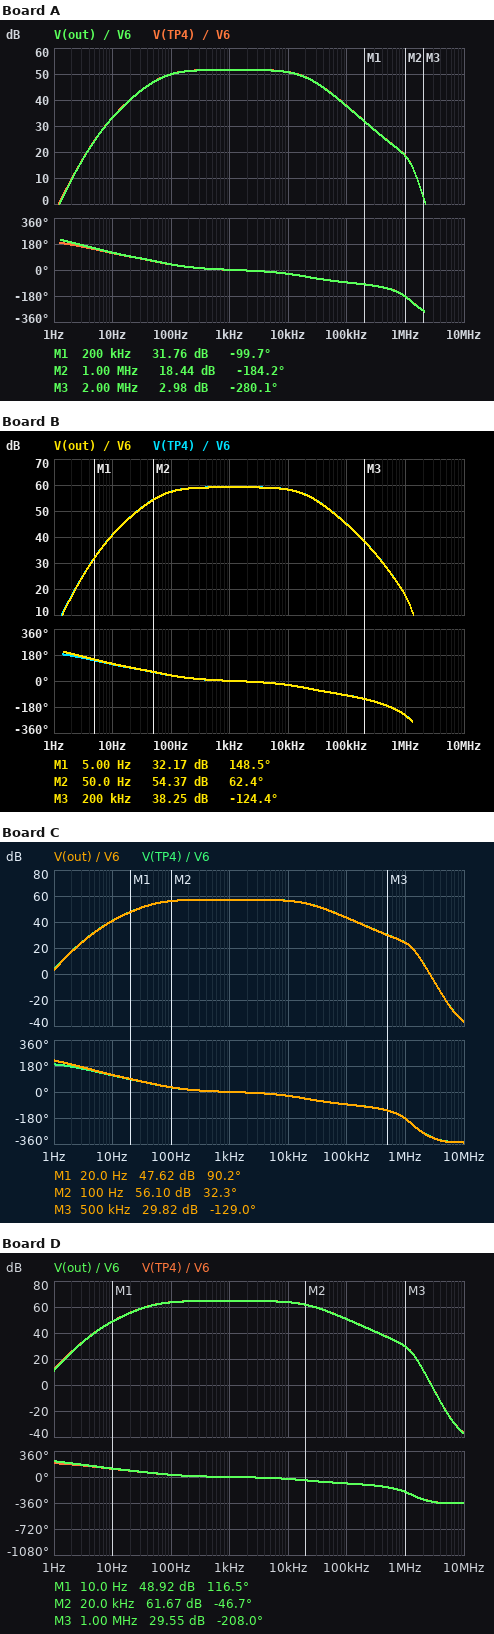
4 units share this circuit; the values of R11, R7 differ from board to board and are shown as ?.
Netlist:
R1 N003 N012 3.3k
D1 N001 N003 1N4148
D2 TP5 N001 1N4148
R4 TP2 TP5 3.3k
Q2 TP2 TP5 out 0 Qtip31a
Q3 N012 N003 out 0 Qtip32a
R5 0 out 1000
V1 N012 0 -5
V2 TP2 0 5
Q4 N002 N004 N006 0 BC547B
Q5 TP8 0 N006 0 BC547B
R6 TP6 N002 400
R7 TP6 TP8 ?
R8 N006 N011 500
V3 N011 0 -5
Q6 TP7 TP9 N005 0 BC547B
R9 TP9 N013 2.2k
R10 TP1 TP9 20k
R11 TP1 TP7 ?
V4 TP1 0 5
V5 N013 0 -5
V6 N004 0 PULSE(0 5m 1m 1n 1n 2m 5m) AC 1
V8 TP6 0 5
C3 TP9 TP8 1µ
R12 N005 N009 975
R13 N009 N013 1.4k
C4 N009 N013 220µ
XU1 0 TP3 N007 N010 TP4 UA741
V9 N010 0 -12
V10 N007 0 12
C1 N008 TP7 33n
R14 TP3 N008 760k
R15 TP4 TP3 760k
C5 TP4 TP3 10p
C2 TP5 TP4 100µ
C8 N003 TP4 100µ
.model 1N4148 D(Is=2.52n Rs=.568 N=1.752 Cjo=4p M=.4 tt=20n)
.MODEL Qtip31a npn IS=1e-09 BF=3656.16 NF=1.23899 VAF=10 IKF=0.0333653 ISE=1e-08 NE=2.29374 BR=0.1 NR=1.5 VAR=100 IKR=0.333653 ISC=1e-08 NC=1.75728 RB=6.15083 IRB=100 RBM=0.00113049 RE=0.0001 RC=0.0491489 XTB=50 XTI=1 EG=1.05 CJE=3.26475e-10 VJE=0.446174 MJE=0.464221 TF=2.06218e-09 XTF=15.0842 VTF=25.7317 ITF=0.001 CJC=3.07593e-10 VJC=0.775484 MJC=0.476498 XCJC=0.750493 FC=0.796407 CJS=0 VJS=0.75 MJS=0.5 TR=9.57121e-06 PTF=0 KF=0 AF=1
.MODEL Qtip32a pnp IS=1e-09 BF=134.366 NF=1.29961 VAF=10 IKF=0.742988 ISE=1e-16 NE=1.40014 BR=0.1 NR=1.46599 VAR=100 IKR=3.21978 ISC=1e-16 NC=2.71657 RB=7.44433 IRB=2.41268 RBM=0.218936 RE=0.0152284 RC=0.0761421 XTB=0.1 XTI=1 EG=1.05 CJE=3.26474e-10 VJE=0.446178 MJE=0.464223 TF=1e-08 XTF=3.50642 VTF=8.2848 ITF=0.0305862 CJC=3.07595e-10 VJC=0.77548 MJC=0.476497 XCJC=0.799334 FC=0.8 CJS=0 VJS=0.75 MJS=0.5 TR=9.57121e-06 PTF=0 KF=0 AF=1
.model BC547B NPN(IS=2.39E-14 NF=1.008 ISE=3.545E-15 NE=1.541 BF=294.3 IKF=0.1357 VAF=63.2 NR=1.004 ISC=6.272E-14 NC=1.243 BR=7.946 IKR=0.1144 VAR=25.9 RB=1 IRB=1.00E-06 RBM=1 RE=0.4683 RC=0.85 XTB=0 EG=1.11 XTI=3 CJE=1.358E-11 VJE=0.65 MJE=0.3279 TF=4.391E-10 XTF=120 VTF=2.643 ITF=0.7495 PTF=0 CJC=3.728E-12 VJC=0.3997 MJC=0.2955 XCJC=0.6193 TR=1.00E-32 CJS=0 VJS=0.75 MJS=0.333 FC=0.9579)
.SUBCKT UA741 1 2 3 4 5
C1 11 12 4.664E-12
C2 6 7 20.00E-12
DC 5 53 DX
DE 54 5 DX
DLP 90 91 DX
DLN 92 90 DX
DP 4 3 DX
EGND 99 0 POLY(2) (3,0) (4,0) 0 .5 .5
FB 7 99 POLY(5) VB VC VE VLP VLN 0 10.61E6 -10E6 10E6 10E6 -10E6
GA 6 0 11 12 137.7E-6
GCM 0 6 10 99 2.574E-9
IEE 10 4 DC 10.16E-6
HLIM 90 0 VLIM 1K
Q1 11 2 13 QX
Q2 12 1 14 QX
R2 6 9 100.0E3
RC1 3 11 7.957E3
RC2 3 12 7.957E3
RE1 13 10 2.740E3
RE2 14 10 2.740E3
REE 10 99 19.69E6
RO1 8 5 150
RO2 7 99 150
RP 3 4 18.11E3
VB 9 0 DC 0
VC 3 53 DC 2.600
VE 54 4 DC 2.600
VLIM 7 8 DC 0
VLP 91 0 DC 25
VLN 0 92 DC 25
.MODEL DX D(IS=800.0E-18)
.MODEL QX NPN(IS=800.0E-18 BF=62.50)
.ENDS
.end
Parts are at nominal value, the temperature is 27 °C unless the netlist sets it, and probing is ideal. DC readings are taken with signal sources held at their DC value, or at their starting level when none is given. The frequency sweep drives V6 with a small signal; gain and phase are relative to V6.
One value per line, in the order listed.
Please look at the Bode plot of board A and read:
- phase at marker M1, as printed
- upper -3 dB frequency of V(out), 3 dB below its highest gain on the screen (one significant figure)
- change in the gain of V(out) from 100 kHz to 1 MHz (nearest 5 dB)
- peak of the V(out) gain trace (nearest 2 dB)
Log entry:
-99.7 deg
20 kHz
-20 dB
52 dB
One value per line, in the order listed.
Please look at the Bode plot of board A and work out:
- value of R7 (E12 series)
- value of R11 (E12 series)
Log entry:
330 Ω
22 kΩ
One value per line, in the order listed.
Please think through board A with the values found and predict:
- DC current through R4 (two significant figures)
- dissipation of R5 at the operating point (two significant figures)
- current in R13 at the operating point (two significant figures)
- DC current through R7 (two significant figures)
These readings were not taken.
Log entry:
1.3 mA
19 µW
170 µA
4.3 mA
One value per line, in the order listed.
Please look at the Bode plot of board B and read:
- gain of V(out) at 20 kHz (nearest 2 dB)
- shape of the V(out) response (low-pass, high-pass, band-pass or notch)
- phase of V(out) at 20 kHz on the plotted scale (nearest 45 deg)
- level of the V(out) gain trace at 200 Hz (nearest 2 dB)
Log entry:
56 dB
band-pass
-45 deg
58 dB
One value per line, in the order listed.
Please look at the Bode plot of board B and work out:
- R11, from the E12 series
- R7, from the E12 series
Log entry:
56 kΩ
330 Ω
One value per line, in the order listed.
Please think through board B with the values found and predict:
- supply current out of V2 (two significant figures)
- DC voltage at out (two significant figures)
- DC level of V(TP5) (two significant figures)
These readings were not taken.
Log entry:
56 mA
140 mV
720 mV
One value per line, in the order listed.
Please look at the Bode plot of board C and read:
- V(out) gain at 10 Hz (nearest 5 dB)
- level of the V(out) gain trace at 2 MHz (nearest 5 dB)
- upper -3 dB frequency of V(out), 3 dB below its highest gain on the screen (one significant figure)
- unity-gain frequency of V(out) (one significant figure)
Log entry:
40 dB
10 dB
20 kHz
3 MHz
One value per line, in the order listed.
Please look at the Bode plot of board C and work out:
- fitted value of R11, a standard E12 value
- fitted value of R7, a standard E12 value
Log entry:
18 kΩ
1 kΩ
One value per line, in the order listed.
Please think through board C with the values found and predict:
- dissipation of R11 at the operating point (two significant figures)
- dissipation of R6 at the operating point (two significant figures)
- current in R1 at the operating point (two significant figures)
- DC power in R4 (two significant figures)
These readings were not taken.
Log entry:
510 µW
7.7 mW
1.4 mA
5.5 mW
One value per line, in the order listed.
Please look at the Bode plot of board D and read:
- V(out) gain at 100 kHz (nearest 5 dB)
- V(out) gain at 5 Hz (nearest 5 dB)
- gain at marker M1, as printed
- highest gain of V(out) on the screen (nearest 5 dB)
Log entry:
50 dB
40 dB
48.92 dB
65 dB
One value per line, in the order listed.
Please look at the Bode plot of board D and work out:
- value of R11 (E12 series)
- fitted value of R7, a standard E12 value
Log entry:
39 kΩ
1.2 kΩ
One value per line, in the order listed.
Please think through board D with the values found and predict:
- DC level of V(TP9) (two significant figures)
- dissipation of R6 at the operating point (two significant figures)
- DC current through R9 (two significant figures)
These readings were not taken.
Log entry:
-4.0 V
7.8 mW
450 µA
